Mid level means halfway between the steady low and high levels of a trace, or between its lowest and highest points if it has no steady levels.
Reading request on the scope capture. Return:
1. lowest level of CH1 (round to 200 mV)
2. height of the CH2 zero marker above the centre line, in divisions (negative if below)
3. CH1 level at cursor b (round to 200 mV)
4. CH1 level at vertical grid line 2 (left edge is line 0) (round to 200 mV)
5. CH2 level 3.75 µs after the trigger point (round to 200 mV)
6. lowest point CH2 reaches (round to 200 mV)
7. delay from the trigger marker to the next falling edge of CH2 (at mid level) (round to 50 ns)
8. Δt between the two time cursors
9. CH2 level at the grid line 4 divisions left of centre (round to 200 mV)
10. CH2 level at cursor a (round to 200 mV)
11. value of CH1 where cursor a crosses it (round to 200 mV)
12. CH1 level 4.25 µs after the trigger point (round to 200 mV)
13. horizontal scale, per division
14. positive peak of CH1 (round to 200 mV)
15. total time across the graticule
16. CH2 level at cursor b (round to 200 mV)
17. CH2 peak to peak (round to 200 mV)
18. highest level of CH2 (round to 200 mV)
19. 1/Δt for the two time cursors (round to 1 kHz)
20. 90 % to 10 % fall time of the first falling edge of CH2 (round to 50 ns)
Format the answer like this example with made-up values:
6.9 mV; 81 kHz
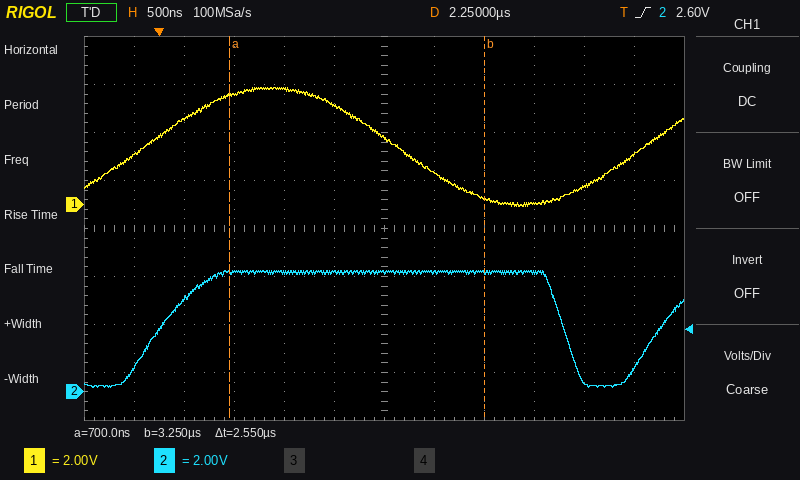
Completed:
0.0 V; -3.4 div; 200 mV; 3.6 V; 5.0 V; 200 mV; 4.05 µs; 2.55 µs; 3.8 V; 5.0 V; 4.6 V; 800 mV; 500 ns; 4.8 V; 6 µs; 5.0 V; 4.8 V; 5.0 V; 392 kHz; 300 ns
